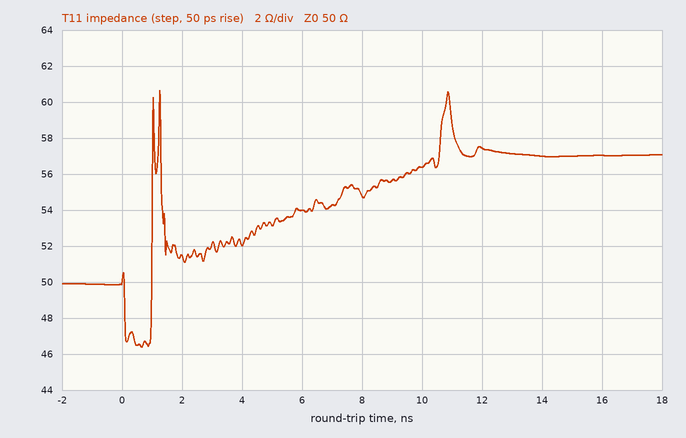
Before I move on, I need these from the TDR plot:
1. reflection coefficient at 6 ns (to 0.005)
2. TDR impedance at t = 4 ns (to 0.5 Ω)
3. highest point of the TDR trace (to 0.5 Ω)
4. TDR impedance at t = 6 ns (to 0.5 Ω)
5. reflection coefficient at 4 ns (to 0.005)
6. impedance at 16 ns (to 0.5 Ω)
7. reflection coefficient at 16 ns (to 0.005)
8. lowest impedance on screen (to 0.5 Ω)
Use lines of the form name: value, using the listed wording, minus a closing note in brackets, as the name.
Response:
reflection coefficient at 6 ns: +0.040
TDR impedance at t = 4 ns: 52.0 Ω
highest point of the TDR trace: 60.5 Ω
TDR impedance at t = 6 ns: 54.0 Ω
reflection coefficient at 4 ns: +0.020
impedance at 16 ns: 57.0 Ω
reflection coefficient at 16 ns: +0.065
lowest impedance on screen: 46.5 Ω
